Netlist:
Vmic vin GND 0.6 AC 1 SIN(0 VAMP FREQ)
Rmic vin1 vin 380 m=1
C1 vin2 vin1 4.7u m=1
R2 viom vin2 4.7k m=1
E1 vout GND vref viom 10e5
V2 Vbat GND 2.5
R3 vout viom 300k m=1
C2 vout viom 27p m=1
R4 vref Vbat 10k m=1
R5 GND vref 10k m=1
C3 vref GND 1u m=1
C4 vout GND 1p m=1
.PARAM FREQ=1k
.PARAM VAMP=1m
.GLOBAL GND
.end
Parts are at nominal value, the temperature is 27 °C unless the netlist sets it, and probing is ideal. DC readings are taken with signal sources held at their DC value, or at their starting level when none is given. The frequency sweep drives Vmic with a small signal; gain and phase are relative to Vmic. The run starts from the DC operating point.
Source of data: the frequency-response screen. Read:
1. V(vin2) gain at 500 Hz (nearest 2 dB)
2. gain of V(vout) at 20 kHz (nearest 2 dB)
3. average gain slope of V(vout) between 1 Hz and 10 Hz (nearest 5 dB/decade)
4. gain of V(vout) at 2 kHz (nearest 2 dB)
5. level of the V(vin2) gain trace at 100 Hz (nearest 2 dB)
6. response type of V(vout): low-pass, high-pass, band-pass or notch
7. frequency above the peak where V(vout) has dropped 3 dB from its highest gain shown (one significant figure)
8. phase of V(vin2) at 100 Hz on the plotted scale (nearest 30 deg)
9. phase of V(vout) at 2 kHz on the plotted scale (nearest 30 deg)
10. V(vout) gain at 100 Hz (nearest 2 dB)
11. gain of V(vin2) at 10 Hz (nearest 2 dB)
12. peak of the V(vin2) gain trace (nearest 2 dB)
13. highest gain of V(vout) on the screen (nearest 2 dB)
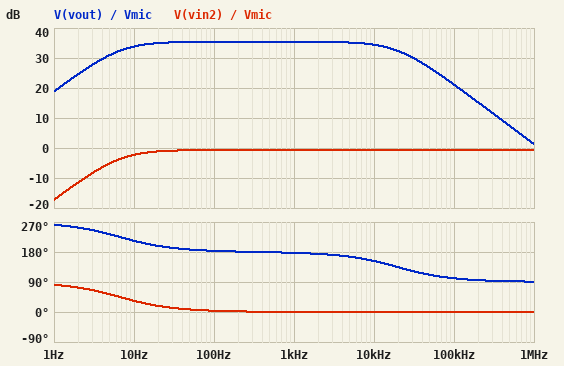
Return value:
0 dB
32 dB
15 dB/decade
36 dB
0 dB
band-pass
20 kHz
0 deg
180 deg
36 dB
-2 dB
0 dB
36 dB
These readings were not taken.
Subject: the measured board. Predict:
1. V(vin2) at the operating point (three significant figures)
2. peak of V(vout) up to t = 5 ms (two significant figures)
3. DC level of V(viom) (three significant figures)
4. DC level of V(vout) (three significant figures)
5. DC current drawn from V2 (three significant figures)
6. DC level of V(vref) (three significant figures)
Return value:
1.25 V
1.3 V
1.25 V
1.25 V
125 µA
1.25 V
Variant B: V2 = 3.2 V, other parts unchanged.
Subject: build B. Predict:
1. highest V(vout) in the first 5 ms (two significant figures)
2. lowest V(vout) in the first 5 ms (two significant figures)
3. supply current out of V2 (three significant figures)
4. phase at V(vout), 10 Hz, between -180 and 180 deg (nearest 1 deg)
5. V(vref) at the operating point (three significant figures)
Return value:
1.7 V
1.5 V
160 µA
-146 deg
1.60 V
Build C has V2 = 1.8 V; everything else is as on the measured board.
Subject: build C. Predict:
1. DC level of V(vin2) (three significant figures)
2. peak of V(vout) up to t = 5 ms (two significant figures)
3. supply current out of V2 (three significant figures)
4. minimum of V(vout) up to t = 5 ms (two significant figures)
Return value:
900 mV
960 mV
90.0 µA
840 mV
